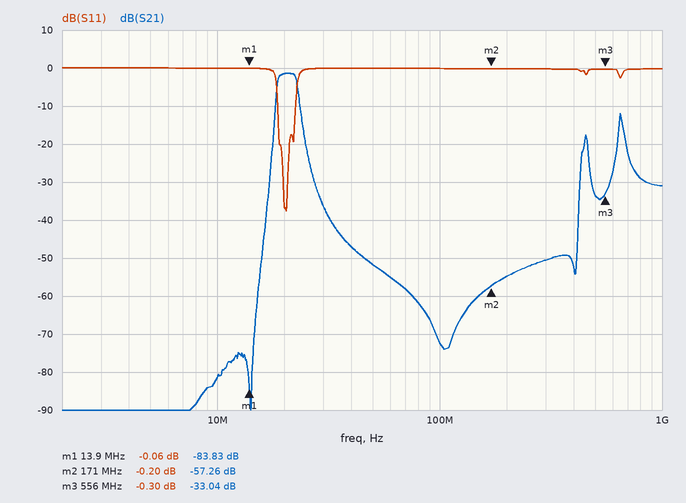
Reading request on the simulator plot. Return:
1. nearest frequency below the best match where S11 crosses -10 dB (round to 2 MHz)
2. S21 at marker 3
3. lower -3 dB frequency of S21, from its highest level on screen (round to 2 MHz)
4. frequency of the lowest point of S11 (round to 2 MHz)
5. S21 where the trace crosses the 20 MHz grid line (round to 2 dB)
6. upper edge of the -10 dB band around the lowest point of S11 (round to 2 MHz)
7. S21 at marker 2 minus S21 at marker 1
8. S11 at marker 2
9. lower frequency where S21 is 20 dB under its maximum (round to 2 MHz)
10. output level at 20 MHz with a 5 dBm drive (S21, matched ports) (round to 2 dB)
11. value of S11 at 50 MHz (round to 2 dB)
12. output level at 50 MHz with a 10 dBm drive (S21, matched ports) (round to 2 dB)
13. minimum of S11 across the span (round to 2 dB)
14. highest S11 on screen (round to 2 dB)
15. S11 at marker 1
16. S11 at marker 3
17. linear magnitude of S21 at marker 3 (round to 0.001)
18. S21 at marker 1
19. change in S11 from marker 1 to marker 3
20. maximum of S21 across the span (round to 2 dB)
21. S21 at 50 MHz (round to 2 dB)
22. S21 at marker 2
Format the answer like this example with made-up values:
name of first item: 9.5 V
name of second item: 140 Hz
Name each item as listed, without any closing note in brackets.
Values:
nearest frequency below the best match where S11 crosses -10 dB: 18 MHz
S21 at marker 3: -33.04 dB
lower -3 dB frequency of S21, from its highest level on screen: 18 MHz
frequency of the lowest point of S11: 20 MHz
S21 where the trace crosses the 20 MHz grid line: -2 dB
upper edge of the -10 dB band around the lowest point of S11: 22 MHz
S21 at marker 2 minus S21 at marker 1: 26.57 dB
S11 at marker 2: -0.20 dB
lower frequency where S21 is 20 dB under its maximum: 18 MHz
output level at 20 MHz with a 5 dBm drive (S21, matched ports): 4 dBm
value of S11 at 50 MHz: 0 dB
output level at 50 MHz with a 10 dBm drive (S21, matched ports): -42 dBm
minimum of S11 across the span: -38 dB
highest S11 on screen: 0 dB
S11 at marker 1: -0.06 dB
S11 at marker 3: -0.30 dB
linear magnitude of S21 at marker 3: 0.022
S21 at marker 1: -83.83 dB
change in S11 from marker 1 to marker 3: -0.24 dB
maximum of S21 across the span: -2 dB
S21 at 50 MHz: -52 dB
S21 at marker 2: -57.26 dB
